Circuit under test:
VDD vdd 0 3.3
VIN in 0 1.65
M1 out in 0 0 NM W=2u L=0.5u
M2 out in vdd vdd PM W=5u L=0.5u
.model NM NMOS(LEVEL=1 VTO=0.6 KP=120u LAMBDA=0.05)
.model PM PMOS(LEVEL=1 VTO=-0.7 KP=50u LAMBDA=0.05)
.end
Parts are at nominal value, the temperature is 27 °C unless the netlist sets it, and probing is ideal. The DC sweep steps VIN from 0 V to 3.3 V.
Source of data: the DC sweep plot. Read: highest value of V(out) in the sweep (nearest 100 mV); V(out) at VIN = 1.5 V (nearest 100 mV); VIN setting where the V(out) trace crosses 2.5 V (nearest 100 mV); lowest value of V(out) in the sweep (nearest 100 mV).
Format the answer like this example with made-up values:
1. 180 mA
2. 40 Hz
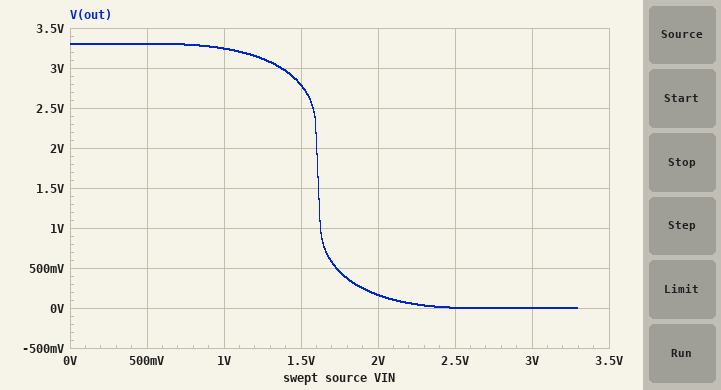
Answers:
1. 3.3 V
2. 2.8 V
3. 1.6 V
4. 0 V
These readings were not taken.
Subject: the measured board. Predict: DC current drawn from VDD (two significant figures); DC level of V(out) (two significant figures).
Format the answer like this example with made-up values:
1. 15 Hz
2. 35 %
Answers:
1. 250 µA
2. 760 mV
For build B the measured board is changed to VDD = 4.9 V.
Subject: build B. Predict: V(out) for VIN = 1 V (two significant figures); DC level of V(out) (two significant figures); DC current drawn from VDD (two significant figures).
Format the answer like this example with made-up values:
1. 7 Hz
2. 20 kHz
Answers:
1. 4.9 V
2. 4.6 V
3. 330 µA
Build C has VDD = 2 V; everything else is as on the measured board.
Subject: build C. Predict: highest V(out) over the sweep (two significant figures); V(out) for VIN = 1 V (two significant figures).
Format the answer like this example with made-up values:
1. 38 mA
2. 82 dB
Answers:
1. 2.0 V
2. 160 mV
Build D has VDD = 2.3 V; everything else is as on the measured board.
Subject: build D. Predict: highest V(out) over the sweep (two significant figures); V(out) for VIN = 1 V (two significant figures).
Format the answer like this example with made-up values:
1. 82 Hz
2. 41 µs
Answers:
1. 2.3 V
2. 2.1 V
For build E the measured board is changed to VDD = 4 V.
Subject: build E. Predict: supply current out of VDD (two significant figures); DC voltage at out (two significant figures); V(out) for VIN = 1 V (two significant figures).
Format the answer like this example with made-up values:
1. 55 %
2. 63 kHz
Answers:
1. 310 µA
2. 3.6 V
3. 4.0 V
